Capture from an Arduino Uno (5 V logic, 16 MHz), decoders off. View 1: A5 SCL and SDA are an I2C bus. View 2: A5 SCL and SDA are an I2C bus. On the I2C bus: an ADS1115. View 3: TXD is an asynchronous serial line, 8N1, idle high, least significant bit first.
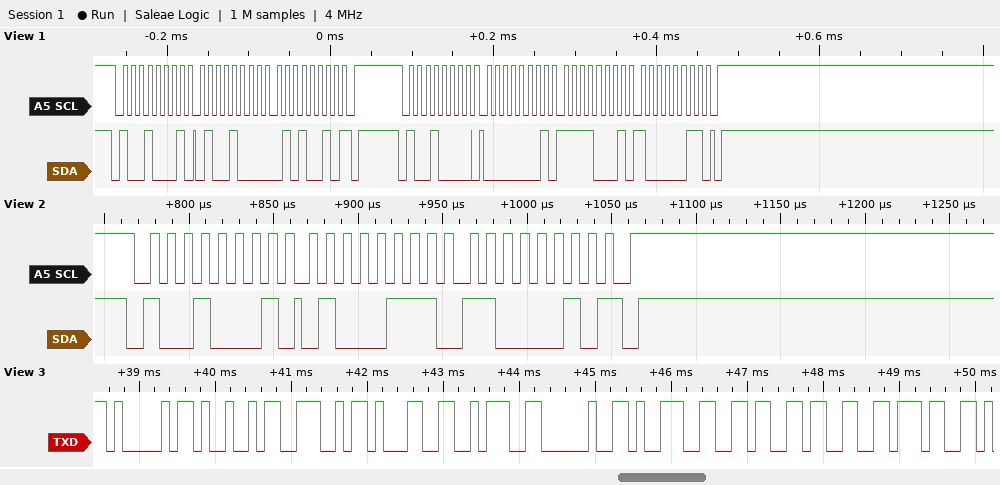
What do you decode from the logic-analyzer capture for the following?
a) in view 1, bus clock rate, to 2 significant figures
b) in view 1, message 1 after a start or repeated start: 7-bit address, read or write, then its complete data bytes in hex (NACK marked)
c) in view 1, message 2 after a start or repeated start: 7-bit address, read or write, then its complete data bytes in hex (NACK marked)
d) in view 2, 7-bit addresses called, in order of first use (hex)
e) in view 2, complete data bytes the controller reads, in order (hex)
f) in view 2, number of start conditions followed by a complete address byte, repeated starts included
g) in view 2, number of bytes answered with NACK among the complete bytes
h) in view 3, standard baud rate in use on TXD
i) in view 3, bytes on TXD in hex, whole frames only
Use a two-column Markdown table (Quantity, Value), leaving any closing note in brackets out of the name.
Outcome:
| Quantity | Value |
|---|---|
| in view 1, bus clock rate, to 2 significant figures | 100 kHz |
| in view 1, message 1 after a start or repeated start: 7-bit address, read or write, then its complete data bytes in hex | 0x48 read: 48 52 NACK |
| in view 1, message 2 after a start or repeated start: 7-bit address, read or write, then its complete data bytes in hex | 0x48 write: 01 F1 83 |
| in view 2, 7-bit addresses called, in order of first use | 0x48 |
| in view 2, complete data bytes the controller reads, in order | 47 C2 |
| in view 2, number of start conditions followed by a complete address byte, repeated starts included | 1 |
| in view 2, number of bytes answered with NACK among the complete bytes | 1 |
| in view 3, standard baud rate in use on TXD | 9600 baud |
| in view 3, bytes on TXD in hex, whole frames only | 41 49 4E 31 3A 20 39 36 33 37 |
